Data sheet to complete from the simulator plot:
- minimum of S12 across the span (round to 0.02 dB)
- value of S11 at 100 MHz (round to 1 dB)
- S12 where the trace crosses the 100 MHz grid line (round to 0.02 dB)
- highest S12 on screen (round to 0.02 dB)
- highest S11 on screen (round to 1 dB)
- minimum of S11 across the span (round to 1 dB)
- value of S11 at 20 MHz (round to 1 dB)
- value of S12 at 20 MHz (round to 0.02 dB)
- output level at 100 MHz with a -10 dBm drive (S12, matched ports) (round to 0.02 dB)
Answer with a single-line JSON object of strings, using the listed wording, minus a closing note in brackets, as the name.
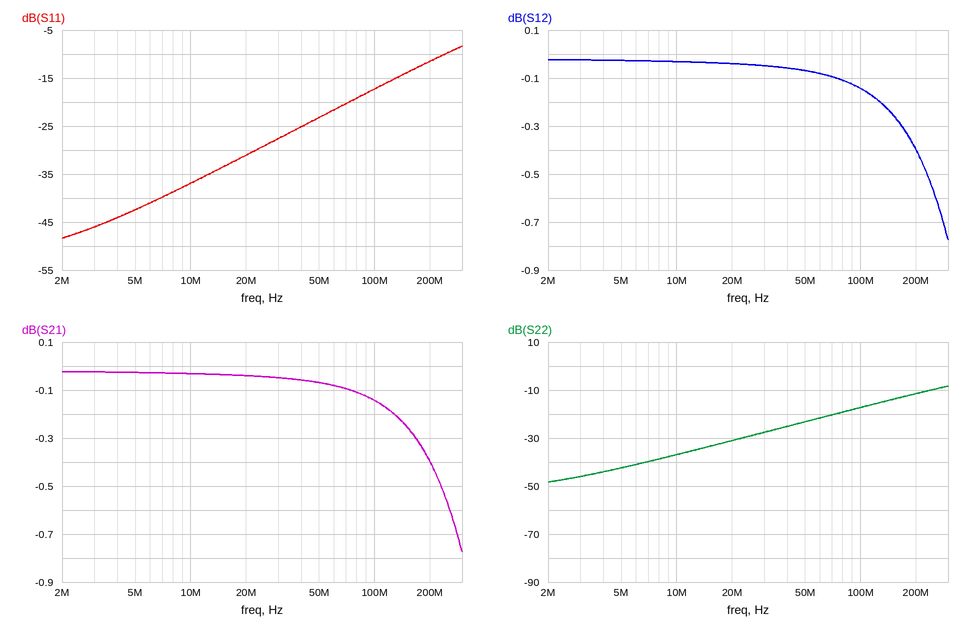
{"minimum of S12 across the span": "-0.78 dB", "value of S11 at 100 MHz": "-17 dB", "S12 where the trace crosses the 100 MHz grid line": "-0.14 dB", "highest S12 on screen": "-0.02 dB", "highest S11 on screen": "-8 dB", "minimum of S11 across the span": "-48 dB", "value of S11 at 20 MHz": "-31 dB", "value of S12 at 20 MHz": "-0.04 dB", "output level at 100 MHz with a -10 dBm drive (S12, matched ports)": "-10.14 dBm"}
